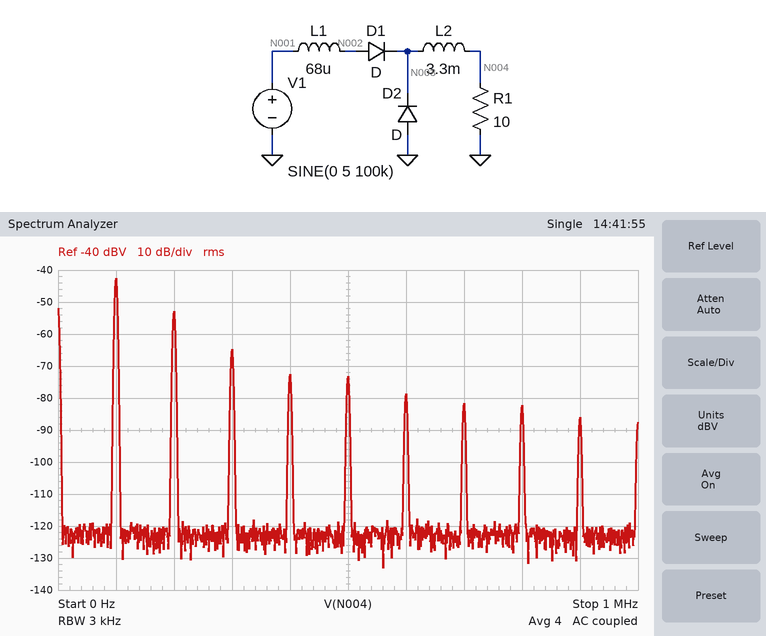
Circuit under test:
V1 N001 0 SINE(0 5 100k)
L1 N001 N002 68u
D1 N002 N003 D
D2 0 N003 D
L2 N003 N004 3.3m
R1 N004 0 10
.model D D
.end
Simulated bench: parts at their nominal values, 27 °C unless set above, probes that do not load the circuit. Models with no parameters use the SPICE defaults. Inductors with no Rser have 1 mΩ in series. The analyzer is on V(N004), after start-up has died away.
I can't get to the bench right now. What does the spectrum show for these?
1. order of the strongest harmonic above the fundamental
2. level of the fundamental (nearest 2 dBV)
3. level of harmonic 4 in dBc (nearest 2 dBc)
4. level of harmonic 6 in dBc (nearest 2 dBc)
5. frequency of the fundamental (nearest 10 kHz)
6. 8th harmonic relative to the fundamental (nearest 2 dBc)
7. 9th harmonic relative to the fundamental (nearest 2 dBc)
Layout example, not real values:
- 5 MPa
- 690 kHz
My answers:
- 2
- -42 dBV
- -30 dBc
- -36 dBc
- 100 kHz
- -40 dBc
- -44 dBc
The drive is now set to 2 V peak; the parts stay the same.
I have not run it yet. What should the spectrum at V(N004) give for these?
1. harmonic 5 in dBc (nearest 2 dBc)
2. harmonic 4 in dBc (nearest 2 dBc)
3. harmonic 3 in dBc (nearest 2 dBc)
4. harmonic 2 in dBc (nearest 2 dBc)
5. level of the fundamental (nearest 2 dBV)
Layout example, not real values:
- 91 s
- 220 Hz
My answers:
- -56 dBc
- -34 dBc
- -48 dBc
- -14 dBc
- -50 dBV
